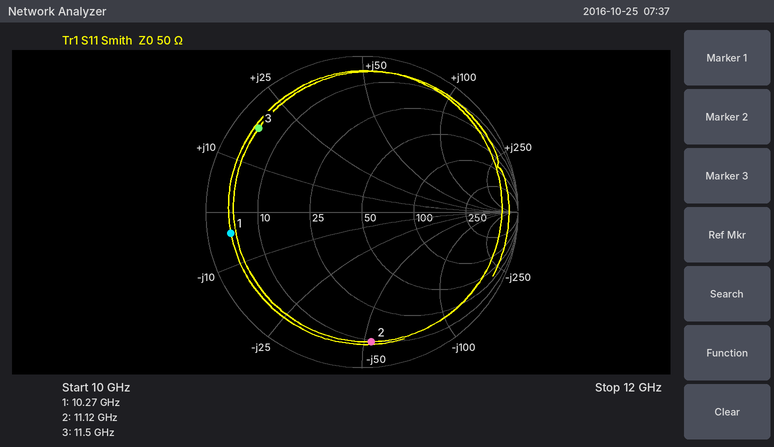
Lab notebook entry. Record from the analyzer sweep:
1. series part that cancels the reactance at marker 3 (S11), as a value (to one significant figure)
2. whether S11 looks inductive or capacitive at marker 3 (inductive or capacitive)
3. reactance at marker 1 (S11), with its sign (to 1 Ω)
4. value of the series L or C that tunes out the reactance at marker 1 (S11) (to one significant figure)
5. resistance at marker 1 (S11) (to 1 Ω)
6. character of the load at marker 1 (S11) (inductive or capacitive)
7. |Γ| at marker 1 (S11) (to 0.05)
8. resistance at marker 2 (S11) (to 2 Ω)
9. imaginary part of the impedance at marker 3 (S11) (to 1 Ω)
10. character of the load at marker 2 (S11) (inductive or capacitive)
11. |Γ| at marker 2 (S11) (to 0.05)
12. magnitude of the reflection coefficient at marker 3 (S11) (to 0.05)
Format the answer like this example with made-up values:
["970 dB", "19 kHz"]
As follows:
["800 fF", "inductive", "-4 Ω", "60 pH", "4 Ω", "capacitive", "0.85", "10 Ω", "+18 Ω", "capacitive", "0.85", "0.85"]
